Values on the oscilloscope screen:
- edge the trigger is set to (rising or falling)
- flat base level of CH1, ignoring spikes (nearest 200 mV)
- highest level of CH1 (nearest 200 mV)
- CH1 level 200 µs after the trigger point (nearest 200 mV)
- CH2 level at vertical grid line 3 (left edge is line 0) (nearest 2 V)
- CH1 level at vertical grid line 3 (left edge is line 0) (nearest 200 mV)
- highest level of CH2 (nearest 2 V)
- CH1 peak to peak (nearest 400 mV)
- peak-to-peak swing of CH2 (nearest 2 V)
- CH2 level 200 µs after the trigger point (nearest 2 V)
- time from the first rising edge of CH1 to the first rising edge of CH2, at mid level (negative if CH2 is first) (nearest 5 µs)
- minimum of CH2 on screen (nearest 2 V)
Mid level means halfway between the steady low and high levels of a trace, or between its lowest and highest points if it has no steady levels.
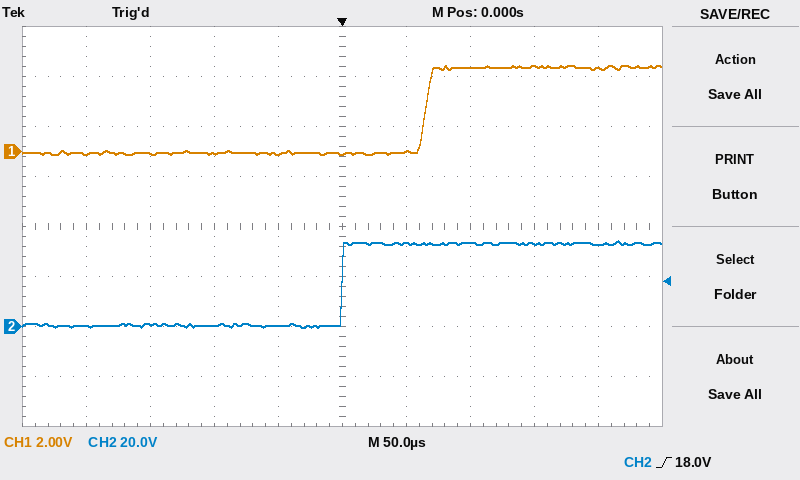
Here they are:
rising
0.0 V
3.4 V
3.4 V
0 V
0.0 V
34 V
3.6 V
34 V
32 V
-65 µs
0 V
